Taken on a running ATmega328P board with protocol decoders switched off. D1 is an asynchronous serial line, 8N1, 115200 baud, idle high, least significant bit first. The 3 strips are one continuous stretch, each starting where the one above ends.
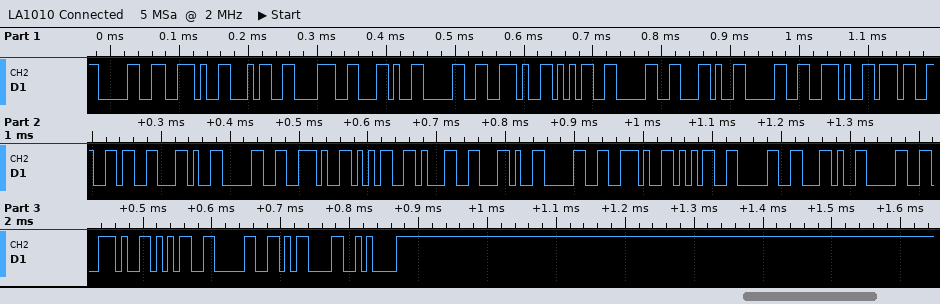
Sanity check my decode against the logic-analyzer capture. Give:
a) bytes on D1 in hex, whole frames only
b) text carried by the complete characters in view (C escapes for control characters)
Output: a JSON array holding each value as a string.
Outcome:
["30 2E 34 38 2C 30 2E 35 30 2C 30 2E 37 36 2C 30 2E 35 31 2C 30 2E 35 30 2C 30 2E 35 30 0D 0A", "\"0.48,0.50,0.76,0.51,0.50,0.50\\r\\n\""]
